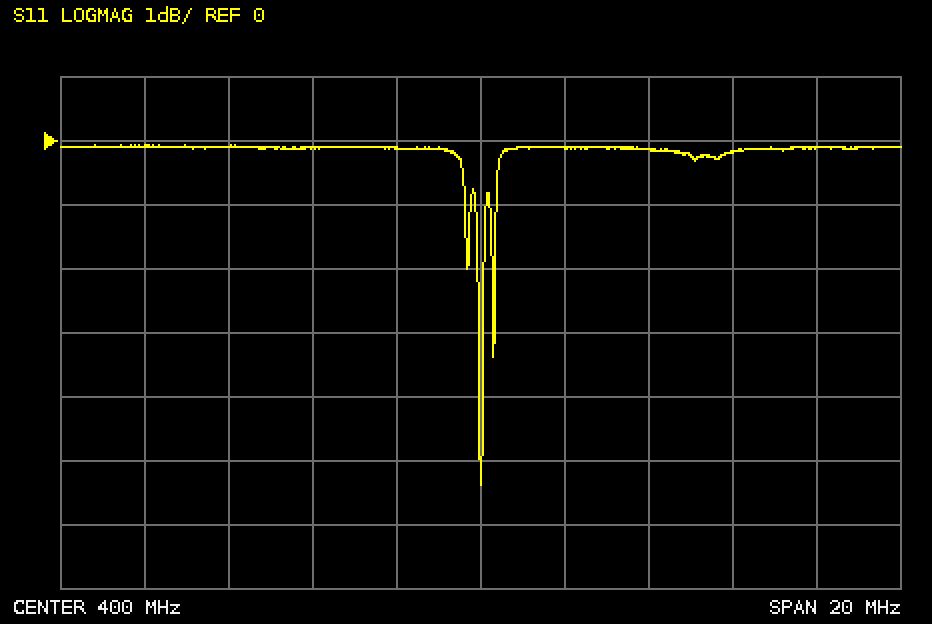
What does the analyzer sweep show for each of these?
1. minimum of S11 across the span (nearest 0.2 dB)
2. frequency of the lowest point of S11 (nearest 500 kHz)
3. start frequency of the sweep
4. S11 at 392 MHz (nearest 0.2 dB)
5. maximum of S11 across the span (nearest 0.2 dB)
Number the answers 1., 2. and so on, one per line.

1. -5.4 dB
2. 400.0 MHz
3. 390 MHz
4. 0.0 dB
5. 0.0 dB
